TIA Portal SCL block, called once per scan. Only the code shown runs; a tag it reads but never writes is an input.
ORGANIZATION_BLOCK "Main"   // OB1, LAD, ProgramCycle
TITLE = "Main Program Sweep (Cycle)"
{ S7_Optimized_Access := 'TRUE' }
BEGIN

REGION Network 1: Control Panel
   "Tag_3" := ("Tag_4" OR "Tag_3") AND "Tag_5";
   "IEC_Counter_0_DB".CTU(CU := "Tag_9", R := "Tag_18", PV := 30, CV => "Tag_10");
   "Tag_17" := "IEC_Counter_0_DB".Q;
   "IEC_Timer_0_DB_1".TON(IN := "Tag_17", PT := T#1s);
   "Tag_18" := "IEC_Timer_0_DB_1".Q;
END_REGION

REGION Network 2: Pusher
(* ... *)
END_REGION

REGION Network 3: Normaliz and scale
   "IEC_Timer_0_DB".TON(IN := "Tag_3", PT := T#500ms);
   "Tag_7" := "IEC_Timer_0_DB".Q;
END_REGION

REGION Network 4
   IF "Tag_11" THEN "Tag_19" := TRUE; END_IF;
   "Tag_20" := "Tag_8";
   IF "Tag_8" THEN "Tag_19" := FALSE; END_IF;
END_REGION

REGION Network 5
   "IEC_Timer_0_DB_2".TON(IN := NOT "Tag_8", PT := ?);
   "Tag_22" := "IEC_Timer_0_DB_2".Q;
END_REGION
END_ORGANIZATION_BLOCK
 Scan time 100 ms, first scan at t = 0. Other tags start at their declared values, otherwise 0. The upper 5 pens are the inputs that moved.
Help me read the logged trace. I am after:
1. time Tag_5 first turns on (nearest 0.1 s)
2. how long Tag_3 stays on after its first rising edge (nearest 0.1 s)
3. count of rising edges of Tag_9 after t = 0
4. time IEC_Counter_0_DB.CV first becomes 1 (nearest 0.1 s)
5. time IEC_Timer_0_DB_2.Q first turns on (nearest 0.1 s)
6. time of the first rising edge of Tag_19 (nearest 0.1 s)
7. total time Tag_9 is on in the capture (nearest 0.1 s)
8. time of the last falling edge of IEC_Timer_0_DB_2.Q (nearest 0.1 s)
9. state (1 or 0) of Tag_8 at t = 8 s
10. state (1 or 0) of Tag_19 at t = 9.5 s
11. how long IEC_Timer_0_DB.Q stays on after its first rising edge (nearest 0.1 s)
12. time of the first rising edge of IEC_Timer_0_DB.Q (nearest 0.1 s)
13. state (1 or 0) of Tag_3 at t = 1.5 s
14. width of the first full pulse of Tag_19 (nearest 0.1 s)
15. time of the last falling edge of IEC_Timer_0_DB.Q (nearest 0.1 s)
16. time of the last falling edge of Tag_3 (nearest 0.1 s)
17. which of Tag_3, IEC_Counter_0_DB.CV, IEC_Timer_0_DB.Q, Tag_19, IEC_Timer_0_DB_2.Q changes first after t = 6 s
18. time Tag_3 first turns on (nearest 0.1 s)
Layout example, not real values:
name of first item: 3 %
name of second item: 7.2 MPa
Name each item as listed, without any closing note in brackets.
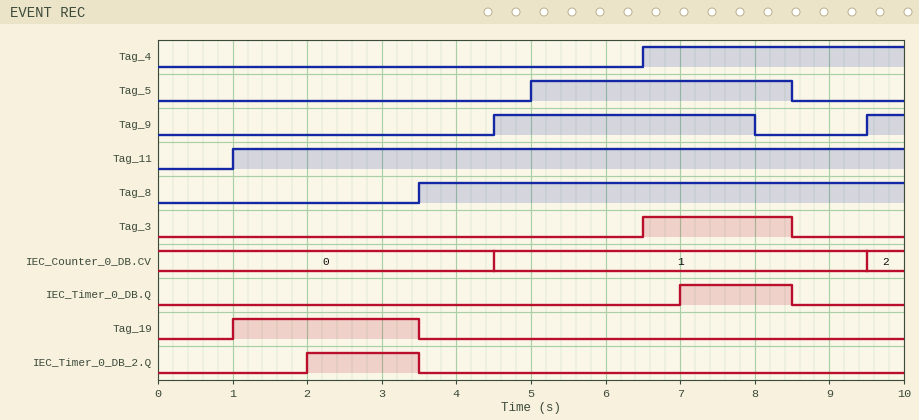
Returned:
time Tag_5 first turns on: 5.0 s
how long Tag_3 stays on after its first rising edge: 2.0 s
count of rising edges of Tag_9 after t = 0: 2
time IEC_Counter_0_DB.CV first becomes 1: 4.5 s
time IEC_Timer_0_DB_2.Q first turns on: 2.0 s
time of the first rising edge of Tag_19: 1.0 s
total time Tag_9 is on in the capture: 4.0 s
time of the last falling edge of IEC_Timer_0_DB_2.Q: 3.5 s
state (1 or 0) of Tag_8 at t = 8 s: 1
state (1 or 0) of Tag_19 at t = 9.5 s: 0
how long IEC_Timer_0_DB.Q stays on after its first rising edge: 1.5 s
time of the first rising edge of IEC_Timer_0_DB.Q: 7.0 s
state (1 or 0) of Tag_3 at t = 1.5 s: 0
width of the first full pulse of Tag_19: 2.5 s
time of the last falling edge of IEC_Timer_0_DB.Q: 8.5 s
time of the last falling edge of Tag_3: 8.5 s
which of Tag_3, IEC_Counter_0_DB.CV, IEC_Timer_0_DB.Q, Tag_19, IEC_Timer_0_DB_2.Q changes first after t = 6 s: Tag_3
time Tag_3 first turns on: 6.5 s
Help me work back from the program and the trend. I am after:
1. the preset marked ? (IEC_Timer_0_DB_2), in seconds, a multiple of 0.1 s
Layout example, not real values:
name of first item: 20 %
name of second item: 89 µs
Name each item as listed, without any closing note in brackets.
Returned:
the preset marked ? (IEC_Timer_0_DB_2), in seconds, a multiple of 0.1 s: 2.0 s
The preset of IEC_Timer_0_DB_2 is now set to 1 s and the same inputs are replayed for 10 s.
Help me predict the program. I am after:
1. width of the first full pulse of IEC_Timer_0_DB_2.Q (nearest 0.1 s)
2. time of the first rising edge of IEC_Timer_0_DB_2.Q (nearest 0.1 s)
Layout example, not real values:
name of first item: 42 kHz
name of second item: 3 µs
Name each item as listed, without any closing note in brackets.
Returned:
width of the first full pulse of IEC_Timer_0_DB_2.Q: 2.5 s
time of the first rising edge of IEC_Timer_0_DB_2.Q: 1.0 s
